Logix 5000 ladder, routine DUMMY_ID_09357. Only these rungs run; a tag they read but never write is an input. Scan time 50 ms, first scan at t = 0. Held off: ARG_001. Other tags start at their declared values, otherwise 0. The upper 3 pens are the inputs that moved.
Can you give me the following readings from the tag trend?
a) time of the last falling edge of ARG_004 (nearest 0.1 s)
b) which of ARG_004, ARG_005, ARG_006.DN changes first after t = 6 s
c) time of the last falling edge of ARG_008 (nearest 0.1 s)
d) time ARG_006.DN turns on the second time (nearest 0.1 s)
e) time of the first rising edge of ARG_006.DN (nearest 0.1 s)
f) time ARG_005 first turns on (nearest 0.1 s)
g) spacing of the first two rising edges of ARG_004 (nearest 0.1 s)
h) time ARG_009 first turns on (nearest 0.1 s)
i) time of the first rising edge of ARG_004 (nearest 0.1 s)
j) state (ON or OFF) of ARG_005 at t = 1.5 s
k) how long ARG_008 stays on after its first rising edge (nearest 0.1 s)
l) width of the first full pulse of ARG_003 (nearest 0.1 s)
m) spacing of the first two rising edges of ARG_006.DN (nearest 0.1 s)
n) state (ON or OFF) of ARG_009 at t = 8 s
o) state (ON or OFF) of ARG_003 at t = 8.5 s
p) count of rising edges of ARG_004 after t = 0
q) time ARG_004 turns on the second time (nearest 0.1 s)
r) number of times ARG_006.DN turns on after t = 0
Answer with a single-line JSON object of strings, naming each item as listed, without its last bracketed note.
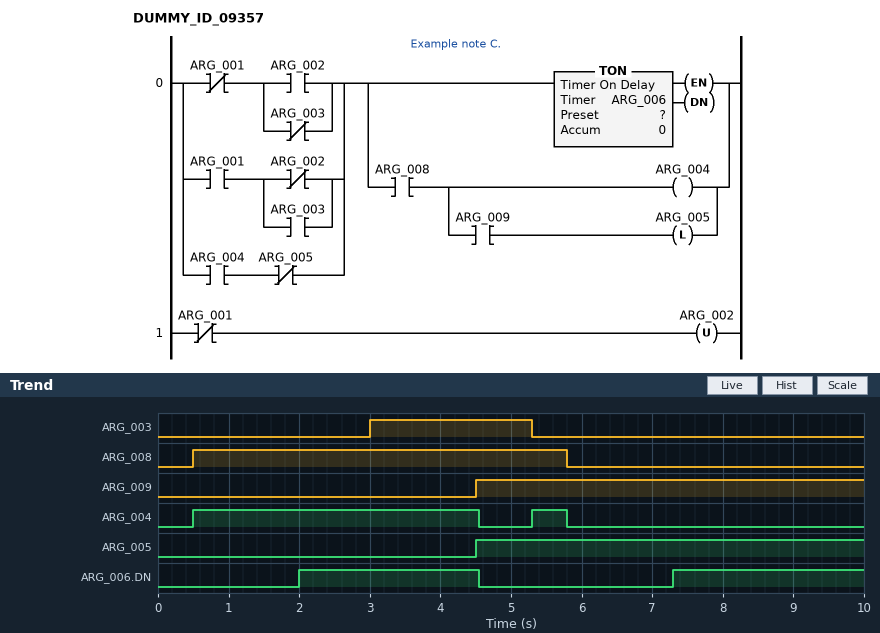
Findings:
{"time of the last falling edge of ARG_004": "5.8 s", "which of ARG_004, ARG_005, ARG_006.DN changes first after t = 6 s": "ARG_006.DN", "time of the last falling edge of ARG_008": "5.8 s", "time ARG_006.DN turns on the second time": "7.3 s", "time of the first rising edge of ARG_006.DN": "2.0 s", "time ARG_005 first turns on": "4.5 s", "spacing of the first two rising edges of ARG_004": "4.8 s", "time ARG_009 first turns on": "4.5 s", "time of the first rising edge of ARG_004": "0.5 s", "state (ON or OFF) of ARG_005 at t = 1.5 s": "OFF", "how long ARG_008 stays on after its first rising edge": "5.3 s", "width of the first full pulse of ARG_003": "2.3 s", "spacing of the first two rising edges of ARG_006.DN": "5.3 s", "state (ON or OFF) of ARG_009 at t = 8 s": "ON", "state (ON or OFF) of ARG_003 at t = 8.5 s": "OFF", "count of rising edges of ARG_004 after t = 0": "2", "time ARG_004 turns on the second time": "5.3 s", "number of times ARG_006.DN turns on after t = 0": "2"}
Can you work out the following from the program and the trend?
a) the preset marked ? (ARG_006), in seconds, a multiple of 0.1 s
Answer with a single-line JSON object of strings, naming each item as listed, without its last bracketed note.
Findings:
{"the preset marked ? (ARG_006), in seconds, a multiple of 0.1 s": "2.0 s"}
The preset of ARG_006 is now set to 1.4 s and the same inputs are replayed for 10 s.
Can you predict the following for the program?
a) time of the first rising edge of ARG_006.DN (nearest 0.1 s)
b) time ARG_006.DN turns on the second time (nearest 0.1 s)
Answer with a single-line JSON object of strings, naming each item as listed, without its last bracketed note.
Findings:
{"time of the first rising edge of ARG_006.DN": "1.4 s", "time ARG_006.DN turns on the second time": "6.7 s"}
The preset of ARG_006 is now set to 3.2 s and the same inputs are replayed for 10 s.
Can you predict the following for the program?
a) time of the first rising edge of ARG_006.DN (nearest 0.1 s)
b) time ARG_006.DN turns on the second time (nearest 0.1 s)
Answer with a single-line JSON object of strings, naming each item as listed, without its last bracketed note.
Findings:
{"time of the first rising edge of ARG_006.DN": "3.2 s", "time ARG_006.DN turns on the second time": "8.5 s"}
